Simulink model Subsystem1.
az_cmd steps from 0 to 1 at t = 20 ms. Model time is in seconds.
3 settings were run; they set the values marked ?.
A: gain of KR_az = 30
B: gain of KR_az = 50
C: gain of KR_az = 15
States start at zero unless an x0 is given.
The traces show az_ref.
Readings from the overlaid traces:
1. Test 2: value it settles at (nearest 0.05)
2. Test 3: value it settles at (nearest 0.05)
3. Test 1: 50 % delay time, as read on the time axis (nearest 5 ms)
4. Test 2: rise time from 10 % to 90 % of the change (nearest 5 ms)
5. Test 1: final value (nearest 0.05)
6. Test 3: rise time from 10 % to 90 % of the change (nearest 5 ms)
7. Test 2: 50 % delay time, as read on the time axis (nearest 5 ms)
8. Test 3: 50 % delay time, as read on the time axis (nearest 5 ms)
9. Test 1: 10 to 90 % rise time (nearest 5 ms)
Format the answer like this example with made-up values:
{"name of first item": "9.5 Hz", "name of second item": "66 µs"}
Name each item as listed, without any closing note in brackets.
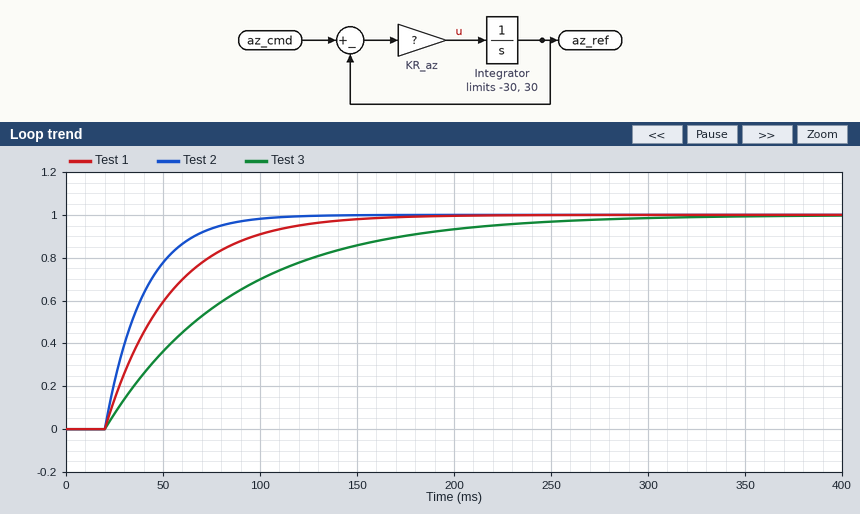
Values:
{"Test 2: value it settles at": "1.00", "Test 3: value it settles at": "1.00", "Test 1: 50 % delay time, as read on the time axis": "45 ms", "Test 2: rise time from 10 % to 90 % of the change": "45 ms", "Test 1: final value": "1.00", "Test 3: rise time from 10 % to 90 % of the change": "145 ms", "Test 2: 50 % delay time, as read on the time axis": "35 ms", "Test 3: 50 % delay time, as read on the time axis": "65 ms", "Test 1: 10 to 90 % rise time": "75 ms"}
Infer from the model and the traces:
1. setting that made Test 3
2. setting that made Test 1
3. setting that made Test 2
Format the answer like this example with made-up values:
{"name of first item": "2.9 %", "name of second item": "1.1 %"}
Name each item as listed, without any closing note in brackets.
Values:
{"setting that made Test 3": "C", "setting that made Test 1": "A", "setting that made Test 2": "B"}
